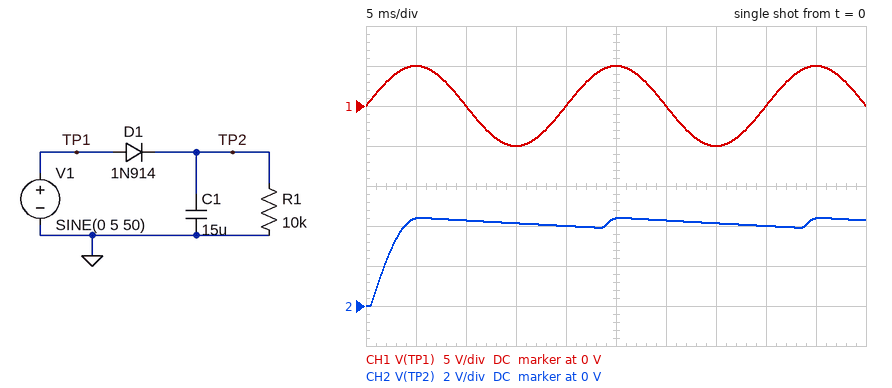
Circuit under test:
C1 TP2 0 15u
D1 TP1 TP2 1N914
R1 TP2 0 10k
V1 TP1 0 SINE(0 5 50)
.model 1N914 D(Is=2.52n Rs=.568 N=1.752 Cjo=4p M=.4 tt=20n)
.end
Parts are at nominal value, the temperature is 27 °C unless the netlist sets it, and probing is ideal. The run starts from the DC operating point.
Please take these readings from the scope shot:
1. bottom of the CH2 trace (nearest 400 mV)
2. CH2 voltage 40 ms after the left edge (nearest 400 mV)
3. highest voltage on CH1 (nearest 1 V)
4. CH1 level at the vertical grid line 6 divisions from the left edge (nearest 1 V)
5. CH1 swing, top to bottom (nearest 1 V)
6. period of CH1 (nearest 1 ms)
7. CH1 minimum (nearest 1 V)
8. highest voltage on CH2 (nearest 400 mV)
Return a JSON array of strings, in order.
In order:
["0 V", "4.0 V", "5 V", "0 V", "10 V", "20 ms", "-5 V", "4.4 V"]
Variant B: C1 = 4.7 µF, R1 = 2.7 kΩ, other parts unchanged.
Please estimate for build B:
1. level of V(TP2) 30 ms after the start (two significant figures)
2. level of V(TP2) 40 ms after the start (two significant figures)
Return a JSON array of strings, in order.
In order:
["3.1 V", "1.4 V"]
